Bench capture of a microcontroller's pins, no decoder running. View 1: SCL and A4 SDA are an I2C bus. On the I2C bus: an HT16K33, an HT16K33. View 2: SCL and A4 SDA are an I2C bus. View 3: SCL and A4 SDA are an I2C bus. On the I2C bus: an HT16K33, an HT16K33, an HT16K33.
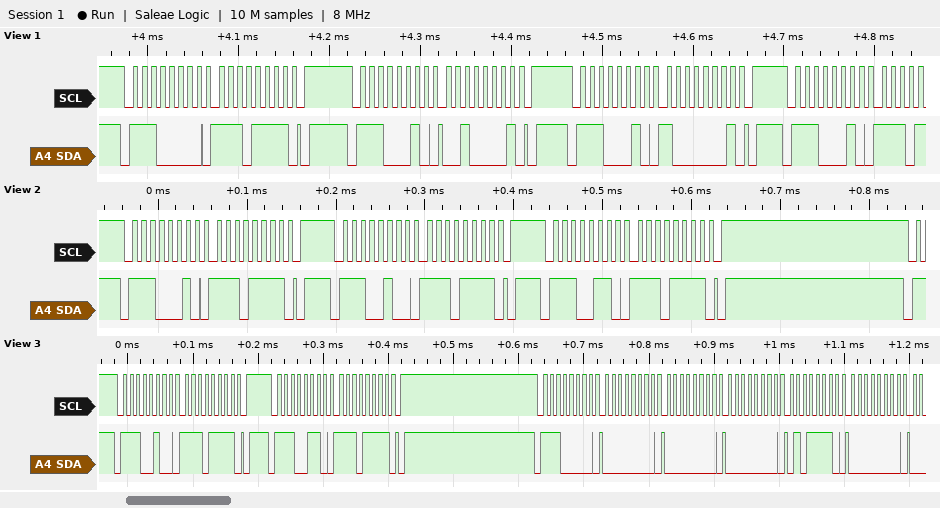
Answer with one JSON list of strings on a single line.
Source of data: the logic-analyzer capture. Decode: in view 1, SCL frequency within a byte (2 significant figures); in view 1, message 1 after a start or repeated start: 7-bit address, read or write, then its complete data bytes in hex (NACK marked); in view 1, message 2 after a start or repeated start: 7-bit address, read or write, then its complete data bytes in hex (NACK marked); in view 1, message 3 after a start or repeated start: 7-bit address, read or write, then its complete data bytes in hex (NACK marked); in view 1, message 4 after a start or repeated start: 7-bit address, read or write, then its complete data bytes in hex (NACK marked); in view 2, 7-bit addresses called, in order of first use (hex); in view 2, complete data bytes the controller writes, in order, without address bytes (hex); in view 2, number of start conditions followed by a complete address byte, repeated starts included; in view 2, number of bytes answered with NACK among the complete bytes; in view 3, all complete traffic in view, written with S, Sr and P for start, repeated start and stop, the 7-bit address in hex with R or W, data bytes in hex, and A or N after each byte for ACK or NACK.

["100 kHz", "0x70 write: EF", "0x71 write: 21", "0x71 write: 81", "0x71 write", "0x71 0x72 0x73", "EF EF EF", "3", "0", "S 72W A EF A P S 73W A EF A P S 70W A 00 A 00 A 00 A 5E A 00 A"]
